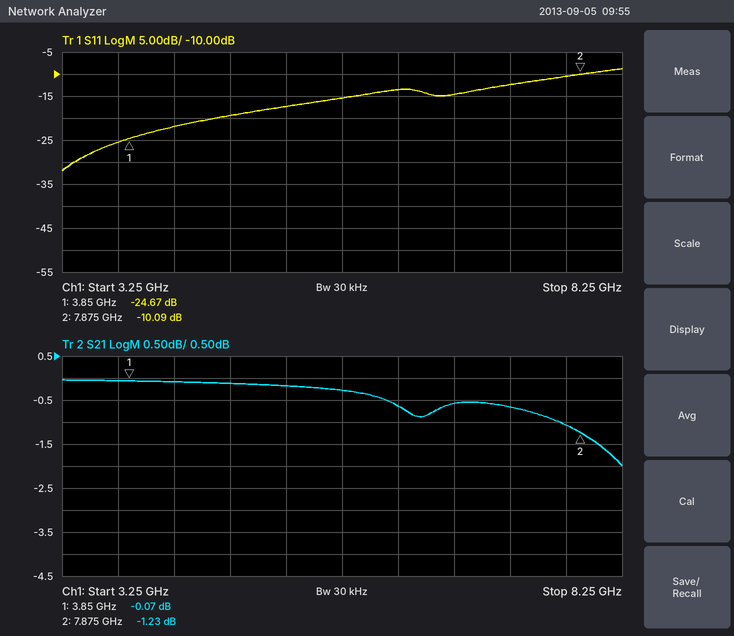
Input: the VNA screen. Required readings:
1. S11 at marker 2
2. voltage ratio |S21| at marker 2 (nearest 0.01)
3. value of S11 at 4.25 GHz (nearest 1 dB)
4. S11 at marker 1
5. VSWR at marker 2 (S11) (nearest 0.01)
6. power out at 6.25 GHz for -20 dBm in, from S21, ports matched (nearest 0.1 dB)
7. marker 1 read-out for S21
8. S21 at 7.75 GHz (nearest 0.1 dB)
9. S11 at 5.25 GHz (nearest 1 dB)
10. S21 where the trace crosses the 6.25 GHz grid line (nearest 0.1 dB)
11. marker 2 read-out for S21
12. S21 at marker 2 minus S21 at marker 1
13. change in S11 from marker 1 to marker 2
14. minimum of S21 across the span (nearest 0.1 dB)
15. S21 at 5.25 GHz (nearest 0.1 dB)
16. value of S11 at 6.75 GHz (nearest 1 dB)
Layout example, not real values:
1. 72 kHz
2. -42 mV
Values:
1. -10.09 dB
2. 0.87
3. -22 dB
4. -24.67 dB
5. 1.91
6. -20.6 dBm
7. -0.07 dB
8. -1.1 dB
9. -17 dB
10. -0.6 dB
11. -1.23 dB
12. -1.16 dB
13. 14.58 dB
14. -2.0 dB
15. -0.2 dB
16. -15 dB
